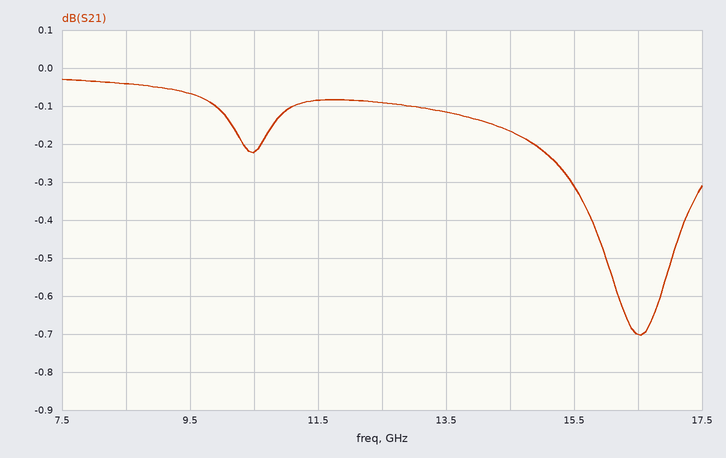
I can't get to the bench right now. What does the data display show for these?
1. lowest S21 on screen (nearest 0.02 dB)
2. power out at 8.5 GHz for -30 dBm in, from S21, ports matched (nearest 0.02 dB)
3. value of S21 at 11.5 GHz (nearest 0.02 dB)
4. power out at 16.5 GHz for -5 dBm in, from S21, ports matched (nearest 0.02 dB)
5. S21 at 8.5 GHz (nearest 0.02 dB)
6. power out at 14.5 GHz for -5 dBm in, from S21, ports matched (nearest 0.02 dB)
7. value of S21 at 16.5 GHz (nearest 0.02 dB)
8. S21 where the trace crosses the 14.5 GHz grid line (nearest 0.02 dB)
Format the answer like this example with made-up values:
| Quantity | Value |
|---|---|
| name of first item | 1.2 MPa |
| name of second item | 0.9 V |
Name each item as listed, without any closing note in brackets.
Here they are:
| Quantity | Value |
|---|---|
| lowest S21 on screen | -0.70 dB |
| power out at 8.5 GHz for -30 dBm in, from S21, ports matched | -30.04 dBm |
| value of S21 at 11.5 GHz | -0.08 dB |
| power out at 16.5 GHz for -5 dBm in, from S21, ports matched | -5.70 dBm |
| S21 at 8.5 GHz | -0.04 dB |
| power out at 14.5 GHz for -5 dBm in, from S21, ports matched | -5.16 dBm |
| value of S21 at 16.5 GHz | -0.70 dB |
| S21 where the trace crosses the 14.5 GHz grid line | -0.16 dB |
